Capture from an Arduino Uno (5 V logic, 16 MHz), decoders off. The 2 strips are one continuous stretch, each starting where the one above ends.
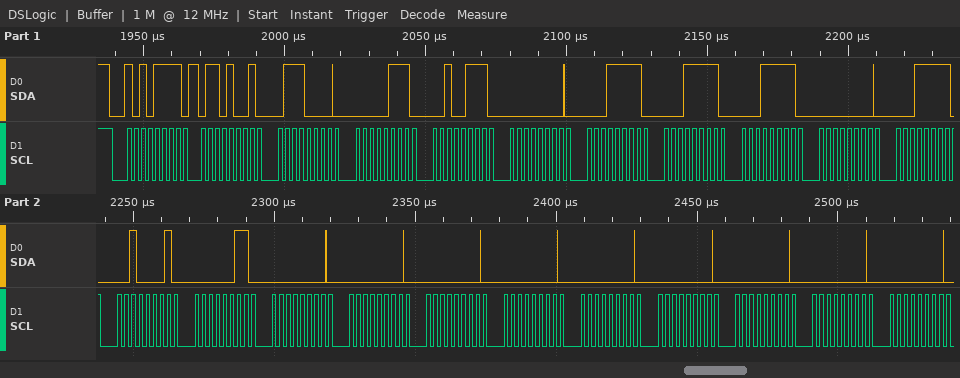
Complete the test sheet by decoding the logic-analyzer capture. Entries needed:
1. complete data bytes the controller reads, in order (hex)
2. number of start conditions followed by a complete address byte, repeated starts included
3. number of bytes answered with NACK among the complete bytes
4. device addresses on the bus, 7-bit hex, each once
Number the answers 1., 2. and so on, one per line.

1. 69 70 07 27 00 1F 1F 1F 00 1F 21 03 00 00 00 00 00 00 00 00 00
2. 1
3. 0
4. 0x57
